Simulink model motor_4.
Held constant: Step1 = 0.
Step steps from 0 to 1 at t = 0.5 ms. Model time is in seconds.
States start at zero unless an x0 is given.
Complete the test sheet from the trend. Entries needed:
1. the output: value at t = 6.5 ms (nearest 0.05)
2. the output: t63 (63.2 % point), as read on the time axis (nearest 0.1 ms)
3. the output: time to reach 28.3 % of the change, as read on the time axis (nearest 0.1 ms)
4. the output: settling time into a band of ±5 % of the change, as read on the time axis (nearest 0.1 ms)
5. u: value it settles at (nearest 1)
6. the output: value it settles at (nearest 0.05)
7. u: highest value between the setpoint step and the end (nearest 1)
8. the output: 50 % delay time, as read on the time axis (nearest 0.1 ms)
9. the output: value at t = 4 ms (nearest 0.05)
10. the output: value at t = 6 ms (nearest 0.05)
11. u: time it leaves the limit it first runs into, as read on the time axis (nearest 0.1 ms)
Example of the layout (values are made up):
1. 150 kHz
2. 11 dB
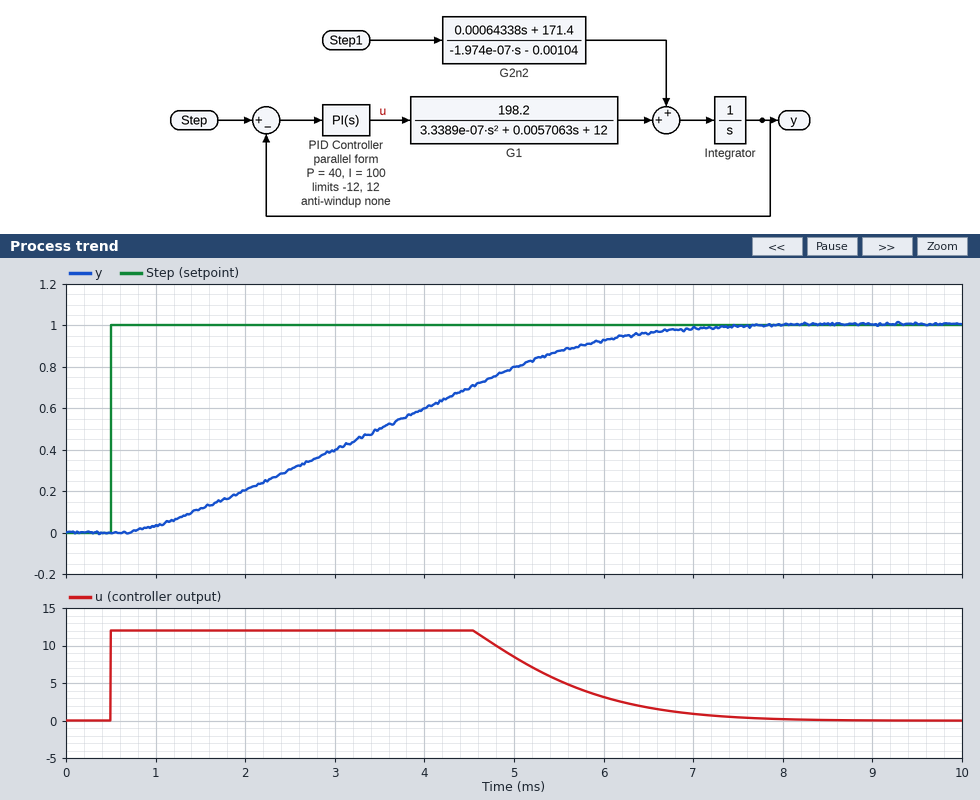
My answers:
1. 0.95
2. 4.2 ms
3. 2.4 ms
4. 6.4 ms
5. 0
6. 1.00
7. 12
8. 3.5 ms
9. 0.60
10. 0.95
11. 4.6 ms
